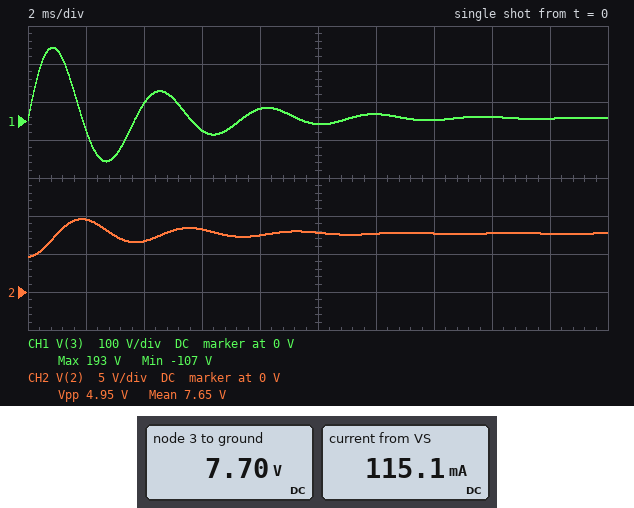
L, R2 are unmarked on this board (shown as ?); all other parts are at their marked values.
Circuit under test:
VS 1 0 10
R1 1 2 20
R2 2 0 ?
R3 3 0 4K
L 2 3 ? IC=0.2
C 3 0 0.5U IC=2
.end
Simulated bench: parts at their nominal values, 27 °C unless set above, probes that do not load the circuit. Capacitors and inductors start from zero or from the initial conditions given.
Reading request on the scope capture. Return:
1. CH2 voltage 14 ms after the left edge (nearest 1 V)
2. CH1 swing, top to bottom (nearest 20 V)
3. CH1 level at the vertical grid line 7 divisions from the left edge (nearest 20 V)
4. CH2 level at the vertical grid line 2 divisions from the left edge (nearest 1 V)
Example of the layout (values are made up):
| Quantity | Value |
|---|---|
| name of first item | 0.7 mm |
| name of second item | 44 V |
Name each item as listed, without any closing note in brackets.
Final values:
| Quantity | Value |
|---|---|
| CH2 voltage 14 ms after the left edge | 8 V |
| CH1 swing, top to bottom | 300 V |
| CH1 level at the vertical grid line 7 divisions from the left edge | 0 V |
| CH2 level at the vertical grid line 2 divisions from the left edge | 7 V |
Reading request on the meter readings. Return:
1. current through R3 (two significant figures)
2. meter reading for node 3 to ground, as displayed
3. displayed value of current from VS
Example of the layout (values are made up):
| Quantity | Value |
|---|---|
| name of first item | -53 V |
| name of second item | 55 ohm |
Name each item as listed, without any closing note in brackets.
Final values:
| Quantity | Value |
|---|---|
| current through R3 | 1.9 mA |
| meter reading for node 3 to ground, as displayed | 7.70 V |
| displayed value of current from VS | 115.1 mA |
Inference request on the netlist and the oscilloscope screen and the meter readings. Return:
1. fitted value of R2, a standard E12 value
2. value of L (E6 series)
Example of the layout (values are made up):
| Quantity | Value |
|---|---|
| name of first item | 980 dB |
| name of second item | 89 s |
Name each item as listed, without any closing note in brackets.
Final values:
| Quantity | Value |
|---|---|
| fitted value of R2, a standard E12 value | 68 Ω |
| value of L | 680 mH |
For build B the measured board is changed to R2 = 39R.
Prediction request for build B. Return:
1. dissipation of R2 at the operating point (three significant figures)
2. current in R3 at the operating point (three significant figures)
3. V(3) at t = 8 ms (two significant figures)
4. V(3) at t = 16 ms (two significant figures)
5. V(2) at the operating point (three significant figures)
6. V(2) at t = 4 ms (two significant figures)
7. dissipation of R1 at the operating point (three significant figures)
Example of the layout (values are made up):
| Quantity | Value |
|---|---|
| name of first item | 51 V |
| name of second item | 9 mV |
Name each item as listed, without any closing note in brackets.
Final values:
| Quantity | Value |
|---|---|
| dissipation of R2 at the operating point | 1.11 W |
| current in R3 at the operating point | 1.65 mA |
| V(3) at t = 8 ms | 31 V |
| V(3) at t = 16 ms | 9.9 V |
| V(2) at the operating point | 6.59 V |
| V(2) at t = 4 ms | 5.7 V |
| dissipation of R1 at the operating point | 582 mW |
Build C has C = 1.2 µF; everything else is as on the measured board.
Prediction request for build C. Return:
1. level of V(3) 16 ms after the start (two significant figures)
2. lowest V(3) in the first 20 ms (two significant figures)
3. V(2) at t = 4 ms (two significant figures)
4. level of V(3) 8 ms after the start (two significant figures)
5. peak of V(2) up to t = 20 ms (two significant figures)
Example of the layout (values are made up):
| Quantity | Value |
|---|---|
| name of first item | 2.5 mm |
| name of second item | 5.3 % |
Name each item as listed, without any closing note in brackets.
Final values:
| Quantity | Value |
|---|---|
| level of V(3) 16 ms after the start | -15 V |
| lowest V(3) in the first 20 ms | -84 V |
| V(2) at t = 4 ms | 8.5 V |
| level of V(3) 8 ms after the start | 43 V |
| peak of V(2) up to t = 20 ms | 9.9 V |
